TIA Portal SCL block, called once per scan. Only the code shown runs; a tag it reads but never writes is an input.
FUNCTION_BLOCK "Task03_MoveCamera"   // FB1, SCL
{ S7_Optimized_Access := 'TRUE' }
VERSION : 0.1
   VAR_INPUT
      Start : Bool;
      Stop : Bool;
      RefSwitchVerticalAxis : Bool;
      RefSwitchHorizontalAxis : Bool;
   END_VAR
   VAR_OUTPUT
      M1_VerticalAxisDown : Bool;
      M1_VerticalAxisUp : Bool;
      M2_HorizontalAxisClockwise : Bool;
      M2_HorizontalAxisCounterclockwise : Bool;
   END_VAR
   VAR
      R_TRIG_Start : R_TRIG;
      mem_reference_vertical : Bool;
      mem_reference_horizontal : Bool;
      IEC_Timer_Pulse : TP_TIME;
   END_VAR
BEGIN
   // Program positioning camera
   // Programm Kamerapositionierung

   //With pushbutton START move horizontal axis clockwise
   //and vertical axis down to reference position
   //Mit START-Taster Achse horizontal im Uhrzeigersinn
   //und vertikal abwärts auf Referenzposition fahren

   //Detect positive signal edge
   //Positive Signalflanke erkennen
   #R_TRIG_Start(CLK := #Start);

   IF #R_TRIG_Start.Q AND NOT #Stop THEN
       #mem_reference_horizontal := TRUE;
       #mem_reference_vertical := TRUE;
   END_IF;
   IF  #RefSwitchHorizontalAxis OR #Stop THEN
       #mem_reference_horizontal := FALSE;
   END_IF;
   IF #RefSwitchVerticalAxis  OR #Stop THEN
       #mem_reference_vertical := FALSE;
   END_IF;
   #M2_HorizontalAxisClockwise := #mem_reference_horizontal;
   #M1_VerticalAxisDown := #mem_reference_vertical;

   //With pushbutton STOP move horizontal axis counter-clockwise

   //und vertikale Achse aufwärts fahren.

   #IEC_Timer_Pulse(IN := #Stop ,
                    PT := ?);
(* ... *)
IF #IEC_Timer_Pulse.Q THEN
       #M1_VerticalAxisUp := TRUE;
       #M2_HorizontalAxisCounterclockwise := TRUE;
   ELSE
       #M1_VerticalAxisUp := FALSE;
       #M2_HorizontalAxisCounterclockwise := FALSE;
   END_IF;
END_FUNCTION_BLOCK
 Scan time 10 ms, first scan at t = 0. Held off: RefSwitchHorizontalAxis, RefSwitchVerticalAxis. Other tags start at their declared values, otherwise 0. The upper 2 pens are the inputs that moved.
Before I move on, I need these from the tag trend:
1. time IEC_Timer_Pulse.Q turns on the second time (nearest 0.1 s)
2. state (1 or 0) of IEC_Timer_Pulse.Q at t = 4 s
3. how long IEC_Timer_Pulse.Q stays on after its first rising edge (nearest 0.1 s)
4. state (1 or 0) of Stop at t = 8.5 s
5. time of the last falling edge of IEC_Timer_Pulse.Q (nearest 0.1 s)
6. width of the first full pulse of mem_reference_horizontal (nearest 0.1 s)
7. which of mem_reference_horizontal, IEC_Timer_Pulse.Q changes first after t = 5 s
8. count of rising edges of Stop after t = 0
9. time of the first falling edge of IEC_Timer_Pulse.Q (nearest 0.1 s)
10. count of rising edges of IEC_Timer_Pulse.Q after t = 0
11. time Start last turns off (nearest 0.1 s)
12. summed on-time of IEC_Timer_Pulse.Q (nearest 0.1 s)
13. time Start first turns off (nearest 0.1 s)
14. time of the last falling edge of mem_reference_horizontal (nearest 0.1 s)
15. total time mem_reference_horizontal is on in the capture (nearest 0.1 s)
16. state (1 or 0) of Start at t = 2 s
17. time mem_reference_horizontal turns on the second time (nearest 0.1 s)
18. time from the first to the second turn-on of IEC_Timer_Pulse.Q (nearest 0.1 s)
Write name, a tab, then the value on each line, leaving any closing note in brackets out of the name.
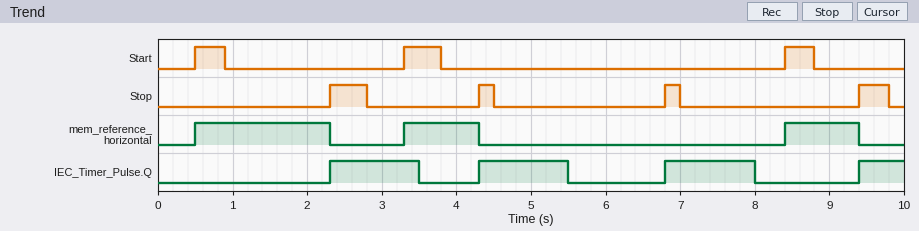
time IEC_Timer_Pulse.Q turns on the second time	4.3 s
state (1 or 0) of IEC_Timer_Pulse.Q at t = 4 s	0
how long IEC_Timer_Pulse.Q stays on after its first rising edge	1.2 s
state (1 or 0) of Stop at t = 8.5 s	0
time of the last falling edge of IEC_Timer_Pulse.Q	8.0 s
width of the first full pulse of mem_reference_horizontal	1.8 s
which of mem_reference_horizontal, IEC_Timer_Pulse.Q changes first after t = 5 s	IEC_Timer_Pulse.Q
count of rising edges of Stop after t = 0	4
time of the first falling edge of IEC_Timer_Pulse.Q	3.5 s
count of rising edges of IEC_Timer_Pulse.Q after t = 0	4
time Start last turns off	8.8 s
summed on-time of IEC_Timer_Pulse.Q	4.2 s
time Start first turns off	0.9 s
time of the last falling edge of mem_reference_horizontal	9.4 s
total time mem_reference_horizontal is on in the capture	3.8 s
state (1 or 0) of Start at t = 2 s	0
time mem_reference_horizontal turns on the second time	3.3 s
time from the first to the second turn-on of IEC_Timer_Pulse.Q	2.0 s
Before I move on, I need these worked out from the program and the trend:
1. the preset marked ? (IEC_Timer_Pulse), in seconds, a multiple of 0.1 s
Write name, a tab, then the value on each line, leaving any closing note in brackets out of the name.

the preset marked ? (IEC_Timer_Pulse), in seconds, a multiple of 0.1 s	1.2 s
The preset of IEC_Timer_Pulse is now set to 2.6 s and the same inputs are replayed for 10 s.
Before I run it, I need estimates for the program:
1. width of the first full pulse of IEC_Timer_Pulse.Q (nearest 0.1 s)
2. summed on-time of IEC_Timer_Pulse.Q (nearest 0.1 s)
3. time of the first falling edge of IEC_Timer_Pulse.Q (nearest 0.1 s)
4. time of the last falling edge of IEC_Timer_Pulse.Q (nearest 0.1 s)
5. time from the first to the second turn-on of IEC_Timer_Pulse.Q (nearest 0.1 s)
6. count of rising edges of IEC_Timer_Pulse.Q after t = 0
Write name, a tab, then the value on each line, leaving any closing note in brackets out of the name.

width of the first full pulse of IEC_Timer_Pulse.Q	2.6 s
summed on-time of IEC_Timer_Pulse.Q	5.2 s
time of the first falling edge of IEC_Timer_Pulse.Q	4.9 s
time of the last falling edge of IEC_Timer_Pulse.Q	9.4 s
time from the first to the second turn-on of IEC_Timer_Pulse.Q	4.5 s
count of rising edges of IEC_Timer_Pulse.Q after t = 0	2
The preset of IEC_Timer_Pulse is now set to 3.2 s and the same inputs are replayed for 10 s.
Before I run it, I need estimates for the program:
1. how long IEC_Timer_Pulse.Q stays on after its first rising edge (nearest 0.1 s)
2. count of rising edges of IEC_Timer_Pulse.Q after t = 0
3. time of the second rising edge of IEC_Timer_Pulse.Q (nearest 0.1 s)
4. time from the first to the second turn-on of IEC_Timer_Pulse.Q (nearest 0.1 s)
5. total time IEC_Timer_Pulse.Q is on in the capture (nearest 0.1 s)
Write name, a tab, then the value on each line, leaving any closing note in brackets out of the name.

how long IEC_Timer_Pulse.Q stays on after its first rising edge	3.2 s
count of rising edges of IEC_Timer_Pulse.Q after t = 0	2
time of the second rising edge of IEC_Timer_Pulse.Q	6.8 s
time from the first to the second turn-on of IEC_Timer_Pulse.Q	4.5 s
total time IEC_Timer_Pulse.Q is on in the capture	6.4 s
